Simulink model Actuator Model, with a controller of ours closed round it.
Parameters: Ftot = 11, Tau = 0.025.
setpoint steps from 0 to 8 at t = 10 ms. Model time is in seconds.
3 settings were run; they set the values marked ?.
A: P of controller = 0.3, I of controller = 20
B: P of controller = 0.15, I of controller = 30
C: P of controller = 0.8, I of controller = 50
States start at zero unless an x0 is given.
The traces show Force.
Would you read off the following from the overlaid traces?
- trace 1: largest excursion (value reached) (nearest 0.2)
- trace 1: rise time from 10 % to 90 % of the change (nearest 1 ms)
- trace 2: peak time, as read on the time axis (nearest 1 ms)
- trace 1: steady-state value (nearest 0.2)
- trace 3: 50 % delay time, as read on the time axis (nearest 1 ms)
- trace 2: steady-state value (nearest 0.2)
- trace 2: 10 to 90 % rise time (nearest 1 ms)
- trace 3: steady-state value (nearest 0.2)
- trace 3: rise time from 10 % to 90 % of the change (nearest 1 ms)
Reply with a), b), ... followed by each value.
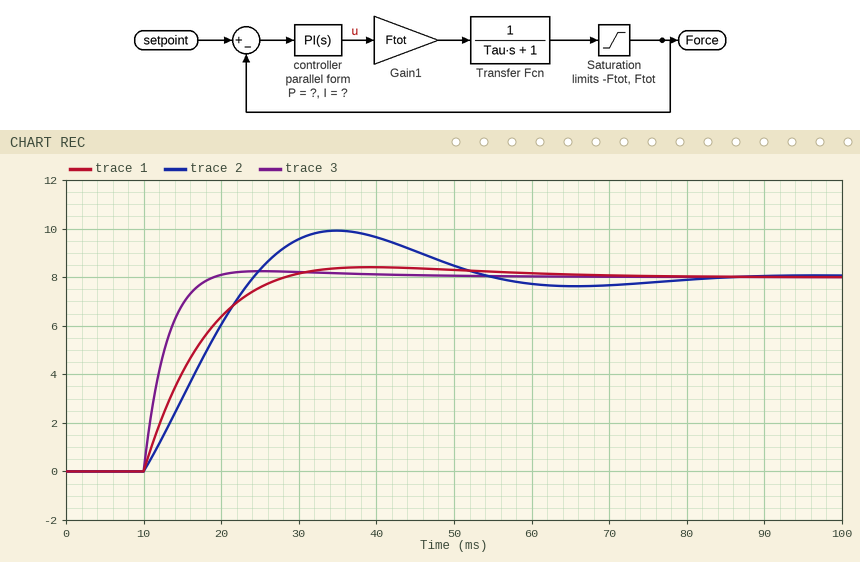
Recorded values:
a) 8.4
b) 12 ms
c) 35 ms
d) 8.0
e) 12 ms
f) 8.0
g) 11 ms
h) 8.0
i) 5 ms
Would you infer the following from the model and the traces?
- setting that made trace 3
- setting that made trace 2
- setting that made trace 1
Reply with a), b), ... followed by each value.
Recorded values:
a) C
b) B
c) A
